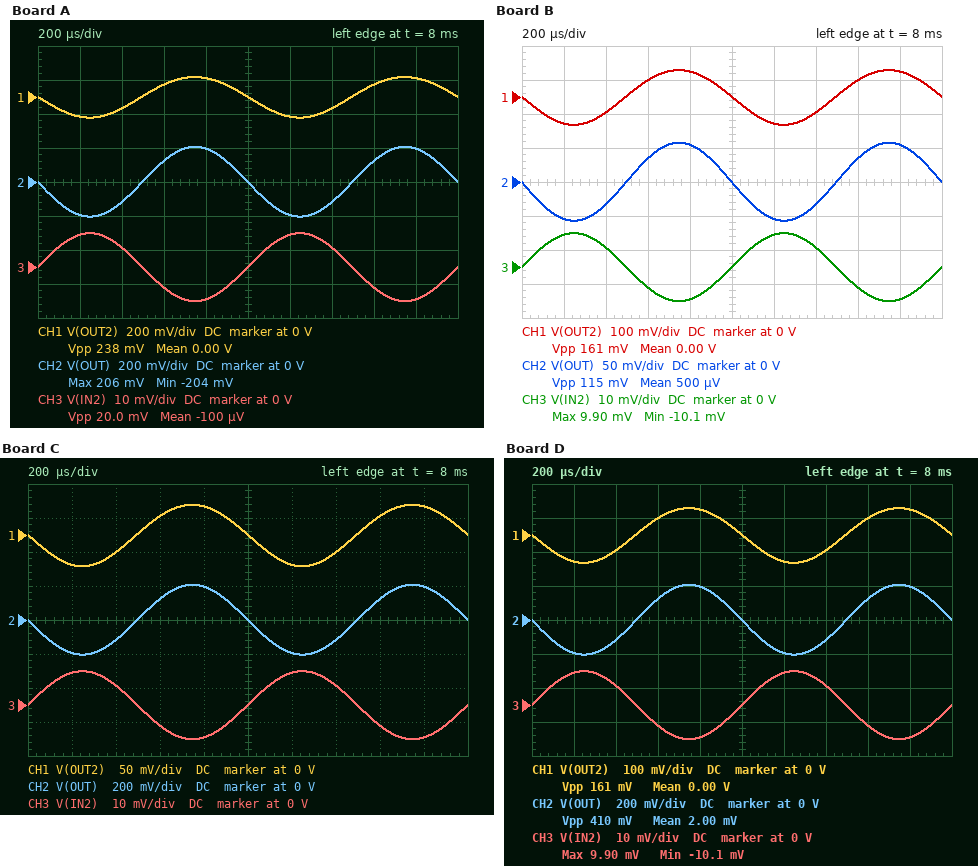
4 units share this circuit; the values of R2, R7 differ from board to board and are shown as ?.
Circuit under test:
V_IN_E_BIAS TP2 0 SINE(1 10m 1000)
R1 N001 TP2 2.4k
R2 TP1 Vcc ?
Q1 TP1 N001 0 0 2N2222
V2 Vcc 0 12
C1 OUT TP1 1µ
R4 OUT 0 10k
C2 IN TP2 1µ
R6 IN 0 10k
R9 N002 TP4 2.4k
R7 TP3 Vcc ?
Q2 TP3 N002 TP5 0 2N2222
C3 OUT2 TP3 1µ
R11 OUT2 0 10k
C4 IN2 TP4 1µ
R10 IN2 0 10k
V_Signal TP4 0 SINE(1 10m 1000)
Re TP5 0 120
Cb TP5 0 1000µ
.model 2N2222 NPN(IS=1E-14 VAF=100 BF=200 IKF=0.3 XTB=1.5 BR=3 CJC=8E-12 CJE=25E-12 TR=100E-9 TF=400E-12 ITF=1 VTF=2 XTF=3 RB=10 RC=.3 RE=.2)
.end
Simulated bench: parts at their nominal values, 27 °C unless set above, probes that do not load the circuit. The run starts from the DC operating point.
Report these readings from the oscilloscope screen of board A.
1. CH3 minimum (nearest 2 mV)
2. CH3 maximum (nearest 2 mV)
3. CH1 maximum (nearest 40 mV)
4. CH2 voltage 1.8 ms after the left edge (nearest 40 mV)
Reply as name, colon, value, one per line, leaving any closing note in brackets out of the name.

CH3 minimum: -10 mV
CH3 maximum: 10 mV
CH1 maximum: 120 mV
CH2 voltage 1.8 ms after the left edge: 200 mV
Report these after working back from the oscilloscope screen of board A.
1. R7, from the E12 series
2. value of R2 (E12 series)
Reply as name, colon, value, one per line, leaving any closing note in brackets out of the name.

R7, from the E12 series: 270 Ω
value of R2: 330 Ω
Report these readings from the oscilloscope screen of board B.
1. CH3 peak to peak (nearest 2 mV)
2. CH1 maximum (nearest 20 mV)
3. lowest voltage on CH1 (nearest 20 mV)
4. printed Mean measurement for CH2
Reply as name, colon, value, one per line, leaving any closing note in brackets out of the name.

CH3 peak to peak: 20 mV
CH1 maximum: 80 mV
lowest voltage on CH1: -80 mV
printed Mean measurement for CH2: 500 µV
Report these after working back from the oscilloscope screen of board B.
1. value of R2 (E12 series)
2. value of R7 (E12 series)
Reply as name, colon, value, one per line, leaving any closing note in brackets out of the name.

value of R2: 82 Ω
value of R7: 180 Ω
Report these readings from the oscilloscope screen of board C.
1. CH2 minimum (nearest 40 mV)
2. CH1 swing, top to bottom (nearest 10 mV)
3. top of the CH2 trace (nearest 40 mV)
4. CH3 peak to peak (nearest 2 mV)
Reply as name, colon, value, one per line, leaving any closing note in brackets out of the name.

CH2 minimum: -200 mV
CH1 swing, top to bottom: 90 mV
top of the CH2 trace: 200 mV
CH3 peak to peak: 20 mV
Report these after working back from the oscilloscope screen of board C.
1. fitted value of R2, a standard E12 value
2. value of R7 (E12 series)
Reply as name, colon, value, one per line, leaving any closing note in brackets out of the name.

fitted value of R2, a standard E12 value: 330 Ω
value of R7: 100 Ω
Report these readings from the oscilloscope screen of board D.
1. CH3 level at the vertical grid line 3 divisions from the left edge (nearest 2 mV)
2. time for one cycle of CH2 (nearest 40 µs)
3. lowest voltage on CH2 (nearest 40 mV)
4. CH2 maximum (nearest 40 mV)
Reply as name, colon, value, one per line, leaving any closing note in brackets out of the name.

CH3 level at the vertical grid line 3 divisions from the left edge: -6 mV
time for one cycle of CH2: 1.00 ms
lowest voltage on CH2: -200 mV
CH2 maximum: 200 mV
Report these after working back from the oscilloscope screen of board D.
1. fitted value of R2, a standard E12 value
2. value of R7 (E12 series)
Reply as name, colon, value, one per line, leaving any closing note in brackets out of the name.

fitted value of R2, a standard E12 value: 330 Ω
value of R7: 180 Ω
